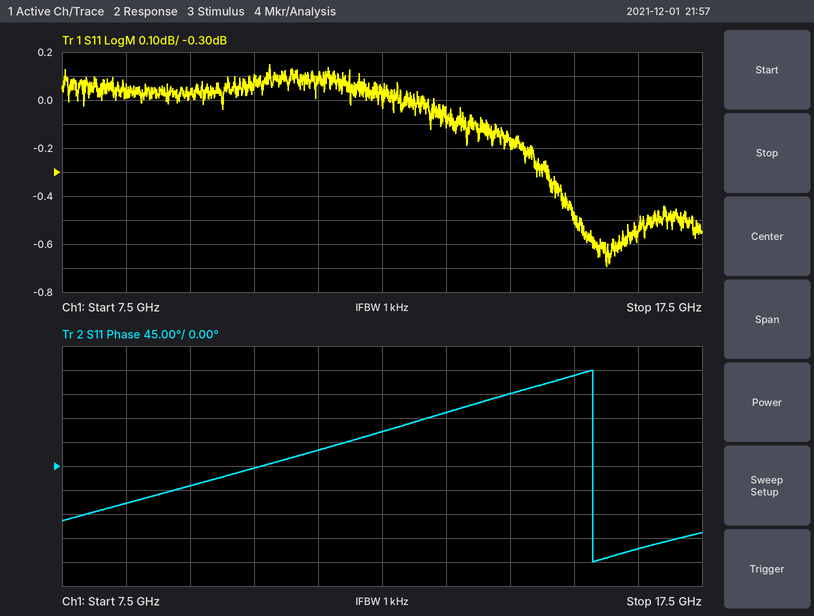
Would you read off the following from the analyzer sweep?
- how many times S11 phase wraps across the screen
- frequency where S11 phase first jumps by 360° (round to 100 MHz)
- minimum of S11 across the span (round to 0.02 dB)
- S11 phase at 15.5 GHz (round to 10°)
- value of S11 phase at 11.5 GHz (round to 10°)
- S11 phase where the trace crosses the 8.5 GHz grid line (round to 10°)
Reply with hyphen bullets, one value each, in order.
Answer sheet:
- 1
- 15.8 GHz
- -0.70 dB
- 170°
- 30°
- -70°
